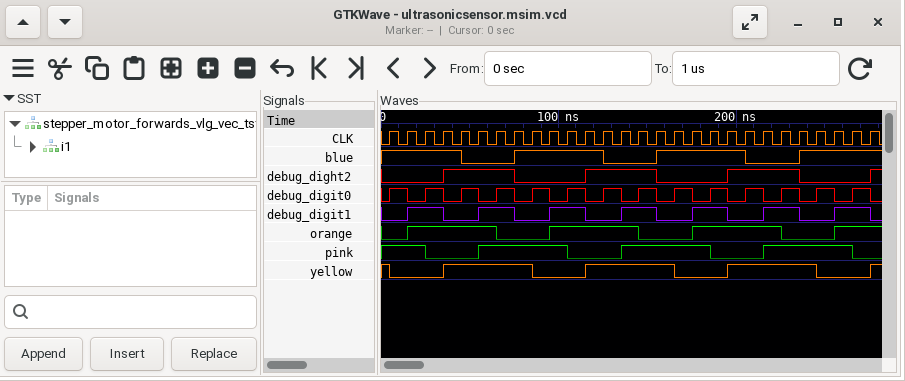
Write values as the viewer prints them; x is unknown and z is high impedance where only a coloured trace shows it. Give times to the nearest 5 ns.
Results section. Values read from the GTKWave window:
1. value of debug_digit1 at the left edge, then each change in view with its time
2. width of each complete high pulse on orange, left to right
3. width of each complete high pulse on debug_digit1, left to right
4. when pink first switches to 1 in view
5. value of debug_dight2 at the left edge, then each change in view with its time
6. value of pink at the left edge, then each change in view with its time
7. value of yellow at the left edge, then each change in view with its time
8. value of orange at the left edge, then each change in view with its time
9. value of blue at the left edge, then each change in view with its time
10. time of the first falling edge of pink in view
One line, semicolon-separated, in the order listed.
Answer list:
0, 1 at 15 ns, 0 at 35 ns, 1 at 55 ns, 0 at 75 ns, 1 at 95 ns, 0 at 115 ns, 1 at 135 ns, 0 at 155 ns, 1 at 175 ns, 0 at 195 ns, 1 at 215 ns, 0 at 235 ns, 1 at 255 ns, 0 at 275 ns; 50 ns, 50 ns, 50 ns; 20 ns, 20 ns, 20 ns, 20 ns, 20 ns, 20 ns, 20 ns; 55 ns; 0, 1 at 35 ns, 0 at 75 ns, 1 at 115 ns, 0 at 155 ns, 1 at 195 ns, 0 at 235 ns, 1 at 275 ns; 1, 0 at 25 ns, 1 at 55 ns, 0 at 105 ns, 1 at 135 ns, 0 at 185 ns, 1 at 215 ns, 0 at 265 ns; 1, 0 at 5 ns, 1 at 35 ns, 0 at 85 ns, 1 at 115 ns, 0 at 165 ns, 1 at 195 ns, 0 at 245 ns, 1 at 275 ns; 0, 1 at 15 ns, 0 at 65 ns, 1 at 95 ns, 0 at 145 ns, 1 at 175 ns, 0 at 225 ns, 1 at 255 ns; 1, 0 at 45 ns, 1 at 75 ns, 0 at 125 ns, 1 at 155 ns, 0 at 205 ns, 1 at 235 ns; 25 ns
